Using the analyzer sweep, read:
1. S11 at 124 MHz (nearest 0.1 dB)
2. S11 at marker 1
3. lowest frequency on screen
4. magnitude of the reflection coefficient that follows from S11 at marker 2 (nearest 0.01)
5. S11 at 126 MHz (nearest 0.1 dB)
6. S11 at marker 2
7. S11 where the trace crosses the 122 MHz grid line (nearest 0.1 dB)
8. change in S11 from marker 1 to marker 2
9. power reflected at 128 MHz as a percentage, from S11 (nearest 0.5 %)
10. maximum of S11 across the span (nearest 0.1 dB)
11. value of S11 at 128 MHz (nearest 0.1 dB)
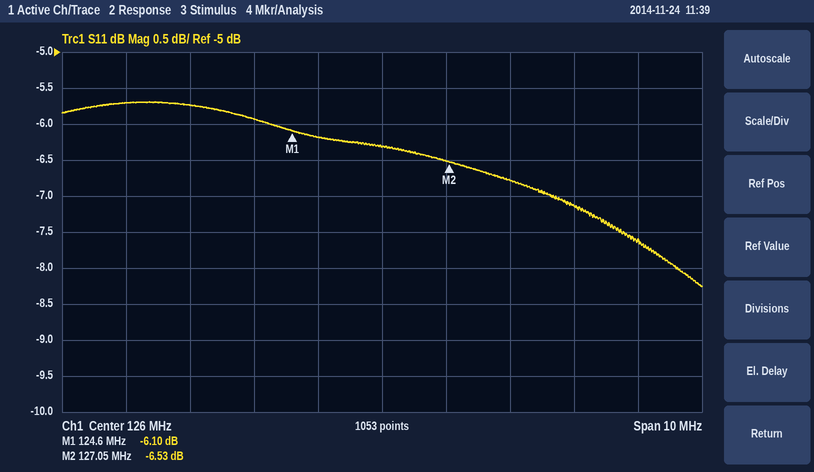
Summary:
-5.9 dB
-6.10 dB
121 MHz
0.47
-6.3 dB
-6.53 dB
-5.7 dB
-0.43 dB
21.0 %
-5.7 dB
-6.8 dB
